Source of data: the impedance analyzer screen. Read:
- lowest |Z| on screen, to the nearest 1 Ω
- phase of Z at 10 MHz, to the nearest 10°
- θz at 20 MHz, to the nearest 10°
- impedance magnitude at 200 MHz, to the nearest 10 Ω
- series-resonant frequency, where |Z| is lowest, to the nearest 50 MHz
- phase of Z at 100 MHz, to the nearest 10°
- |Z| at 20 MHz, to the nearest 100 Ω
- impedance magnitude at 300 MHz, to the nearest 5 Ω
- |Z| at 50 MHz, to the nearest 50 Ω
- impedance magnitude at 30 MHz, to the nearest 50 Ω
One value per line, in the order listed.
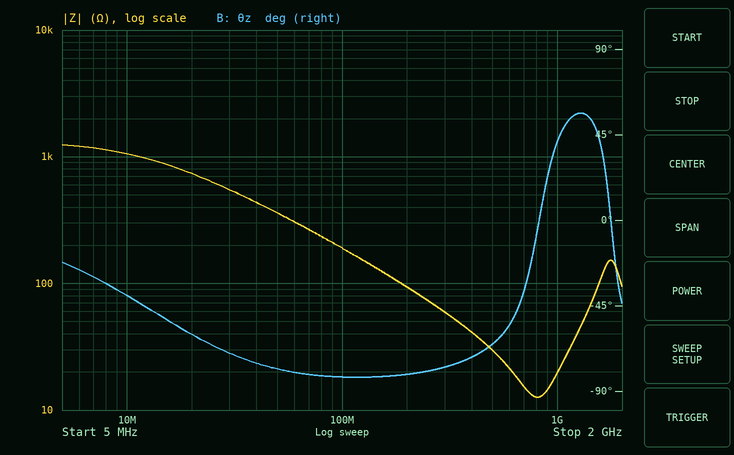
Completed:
13 Ω
-40°
-60°
90 Ω
800 MHz
-80°
700 Ω
60 Ω
350 Ω
550 Ω
